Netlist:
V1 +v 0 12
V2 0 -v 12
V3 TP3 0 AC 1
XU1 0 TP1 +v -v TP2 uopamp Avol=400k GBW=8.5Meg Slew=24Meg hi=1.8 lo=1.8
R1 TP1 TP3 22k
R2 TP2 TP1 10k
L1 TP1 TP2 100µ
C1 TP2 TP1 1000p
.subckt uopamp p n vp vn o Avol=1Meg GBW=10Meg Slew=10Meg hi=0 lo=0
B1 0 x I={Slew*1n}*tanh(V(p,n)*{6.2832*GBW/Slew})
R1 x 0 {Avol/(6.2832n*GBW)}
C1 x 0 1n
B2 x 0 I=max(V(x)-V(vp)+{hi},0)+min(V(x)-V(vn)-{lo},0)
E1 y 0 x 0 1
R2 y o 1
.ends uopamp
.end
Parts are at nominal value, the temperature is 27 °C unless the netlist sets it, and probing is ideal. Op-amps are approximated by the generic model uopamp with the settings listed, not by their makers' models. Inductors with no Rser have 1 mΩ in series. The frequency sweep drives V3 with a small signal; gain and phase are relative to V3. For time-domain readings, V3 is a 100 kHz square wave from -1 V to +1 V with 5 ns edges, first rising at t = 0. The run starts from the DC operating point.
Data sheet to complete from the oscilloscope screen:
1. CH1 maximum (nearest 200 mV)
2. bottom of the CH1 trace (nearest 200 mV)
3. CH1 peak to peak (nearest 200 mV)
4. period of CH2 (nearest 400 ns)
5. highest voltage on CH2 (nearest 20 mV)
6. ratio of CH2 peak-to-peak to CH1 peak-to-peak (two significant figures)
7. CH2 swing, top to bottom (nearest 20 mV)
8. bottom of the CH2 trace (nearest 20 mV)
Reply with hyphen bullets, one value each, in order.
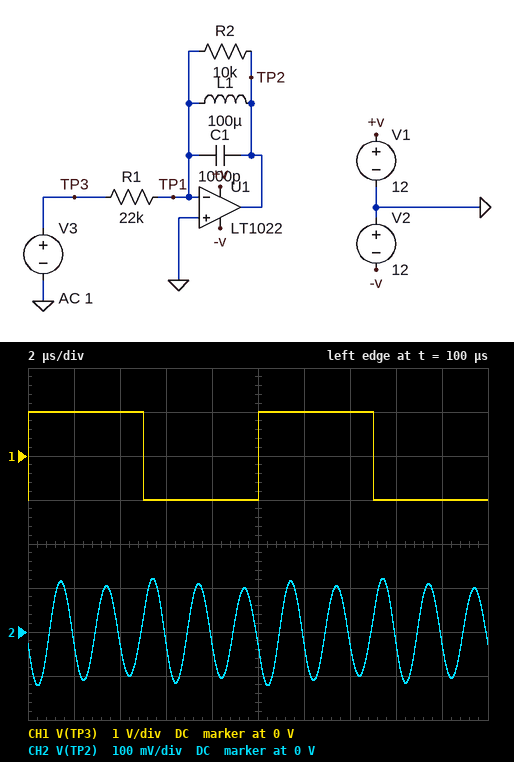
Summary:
- 1.0 V
- -1.0 V
- 2.0 V
- 2.0 µs
- 120 mV
- 0.12
- 240 mV
- -120 mV
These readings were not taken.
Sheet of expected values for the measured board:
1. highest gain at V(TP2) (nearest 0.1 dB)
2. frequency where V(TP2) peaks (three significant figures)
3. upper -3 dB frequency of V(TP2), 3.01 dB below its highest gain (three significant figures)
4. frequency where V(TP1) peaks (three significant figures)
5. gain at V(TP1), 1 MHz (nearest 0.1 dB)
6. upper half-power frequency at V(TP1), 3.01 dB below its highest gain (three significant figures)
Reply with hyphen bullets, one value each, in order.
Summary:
- -6.9 dB
- 503 kHz
- 511 kHz
- 503 kHz
- -58.9 dB
- 511 kHz
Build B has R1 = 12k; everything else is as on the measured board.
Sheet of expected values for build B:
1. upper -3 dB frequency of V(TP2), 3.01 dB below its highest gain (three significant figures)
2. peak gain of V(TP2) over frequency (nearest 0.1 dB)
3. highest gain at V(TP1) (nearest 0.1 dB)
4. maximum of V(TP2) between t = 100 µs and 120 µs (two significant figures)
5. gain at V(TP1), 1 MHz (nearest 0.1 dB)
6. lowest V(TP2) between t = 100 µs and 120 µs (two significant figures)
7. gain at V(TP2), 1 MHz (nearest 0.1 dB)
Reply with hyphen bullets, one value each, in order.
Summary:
- 511 kHz
- -1.6 dB
- -26.2 dB
- 220 mV
- -53.7 dB
- -220 mV
- -35.1 dB
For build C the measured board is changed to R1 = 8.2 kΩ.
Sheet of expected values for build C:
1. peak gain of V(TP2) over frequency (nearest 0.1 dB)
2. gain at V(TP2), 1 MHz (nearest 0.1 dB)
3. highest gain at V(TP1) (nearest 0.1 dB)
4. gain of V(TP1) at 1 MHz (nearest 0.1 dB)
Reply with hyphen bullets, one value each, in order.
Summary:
- 1.7 dB
- -31.8 dB
- -22.9 dB
- -50.4 dB
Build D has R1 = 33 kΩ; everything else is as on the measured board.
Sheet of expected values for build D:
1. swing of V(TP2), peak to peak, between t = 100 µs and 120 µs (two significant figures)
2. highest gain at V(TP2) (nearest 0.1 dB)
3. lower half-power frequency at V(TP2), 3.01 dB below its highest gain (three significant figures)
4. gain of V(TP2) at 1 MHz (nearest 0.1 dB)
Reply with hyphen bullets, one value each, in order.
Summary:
- 160 mV
- -10.4 dB
- 495 kHz
- -43.9 dB
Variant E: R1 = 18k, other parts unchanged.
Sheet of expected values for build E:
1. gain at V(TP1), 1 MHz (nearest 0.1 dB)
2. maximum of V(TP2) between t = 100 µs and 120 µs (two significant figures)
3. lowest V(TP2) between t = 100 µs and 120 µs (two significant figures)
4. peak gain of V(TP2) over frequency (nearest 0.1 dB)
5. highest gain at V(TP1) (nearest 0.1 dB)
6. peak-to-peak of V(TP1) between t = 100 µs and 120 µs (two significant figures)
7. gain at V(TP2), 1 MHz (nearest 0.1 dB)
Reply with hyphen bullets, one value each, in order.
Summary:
- -57.2 dB
- 150 mV
- -150 mV
- -5.1 dB
- -29.7 dB
- 17 mV
- -38.6 dB
